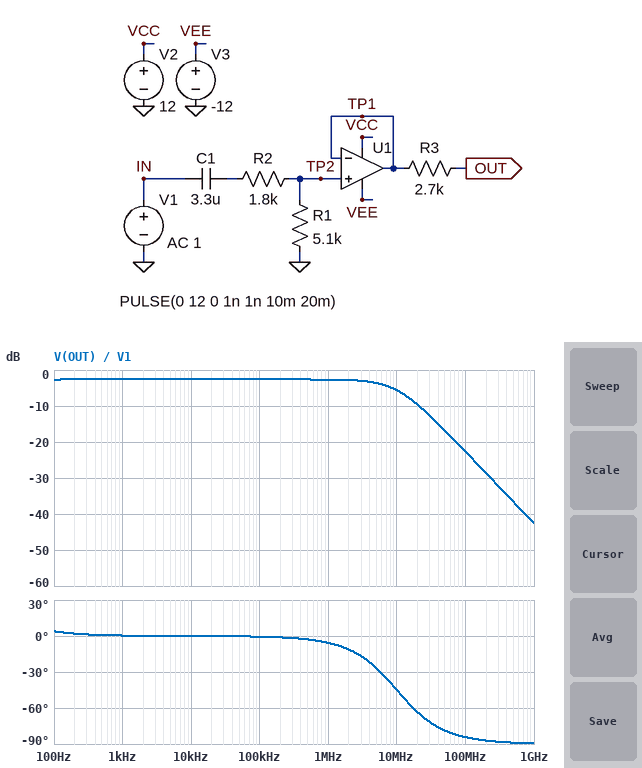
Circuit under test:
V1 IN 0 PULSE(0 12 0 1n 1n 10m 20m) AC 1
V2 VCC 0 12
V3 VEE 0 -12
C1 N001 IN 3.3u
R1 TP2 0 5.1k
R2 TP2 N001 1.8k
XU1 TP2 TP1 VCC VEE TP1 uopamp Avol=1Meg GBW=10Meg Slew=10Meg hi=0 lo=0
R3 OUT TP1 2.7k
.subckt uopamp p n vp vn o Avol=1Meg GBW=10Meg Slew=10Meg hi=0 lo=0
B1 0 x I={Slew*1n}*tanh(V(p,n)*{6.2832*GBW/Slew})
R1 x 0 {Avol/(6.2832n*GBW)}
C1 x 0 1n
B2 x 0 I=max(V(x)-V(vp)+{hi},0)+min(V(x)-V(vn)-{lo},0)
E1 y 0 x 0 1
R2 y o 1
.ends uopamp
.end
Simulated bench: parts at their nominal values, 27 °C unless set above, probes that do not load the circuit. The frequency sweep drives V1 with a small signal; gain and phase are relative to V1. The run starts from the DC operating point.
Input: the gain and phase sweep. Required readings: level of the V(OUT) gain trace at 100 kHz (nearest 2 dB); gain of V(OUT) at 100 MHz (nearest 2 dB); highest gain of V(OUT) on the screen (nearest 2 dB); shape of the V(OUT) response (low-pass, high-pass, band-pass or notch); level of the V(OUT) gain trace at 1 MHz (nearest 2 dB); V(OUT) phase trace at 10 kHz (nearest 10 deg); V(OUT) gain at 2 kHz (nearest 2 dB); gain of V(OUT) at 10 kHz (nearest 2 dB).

-2 dB
-22 dB
-2 dB
low-pass
-2 dB
0 deg
-2 dB
-2 dB
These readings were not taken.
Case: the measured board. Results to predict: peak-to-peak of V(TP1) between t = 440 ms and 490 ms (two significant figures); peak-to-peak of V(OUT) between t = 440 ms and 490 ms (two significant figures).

11 V
11 V
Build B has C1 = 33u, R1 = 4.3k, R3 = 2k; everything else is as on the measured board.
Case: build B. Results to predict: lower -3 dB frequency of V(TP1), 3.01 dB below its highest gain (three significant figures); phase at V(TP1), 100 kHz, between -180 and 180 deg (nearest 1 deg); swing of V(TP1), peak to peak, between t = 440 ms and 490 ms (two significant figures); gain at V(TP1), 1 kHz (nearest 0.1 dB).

791 mHz
-1 deg
8.8 V
-3.0 dB
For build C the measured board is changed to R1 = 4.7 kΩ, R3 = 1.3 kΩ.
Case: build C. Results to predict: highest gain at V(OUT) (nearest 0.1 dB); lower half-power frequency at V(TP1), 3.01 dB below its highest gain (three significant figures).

-2.8 dB
7.42 Hz
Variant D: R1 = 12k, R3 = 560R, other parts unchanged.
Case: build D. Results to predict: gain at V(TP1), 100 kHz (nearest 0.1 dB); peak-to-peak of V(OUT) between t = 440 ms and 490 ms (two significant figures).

-1.2 dB
12 V
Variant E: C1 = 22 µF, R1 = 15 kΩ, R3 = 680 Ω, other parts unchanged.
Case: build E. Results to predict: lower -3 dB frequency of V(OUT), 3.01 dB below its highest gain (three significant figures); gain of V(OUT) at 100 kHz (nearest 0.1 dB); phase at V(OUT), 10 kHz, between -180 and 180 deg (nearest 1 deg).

431 mHz
-1.0 dB
0 deg
